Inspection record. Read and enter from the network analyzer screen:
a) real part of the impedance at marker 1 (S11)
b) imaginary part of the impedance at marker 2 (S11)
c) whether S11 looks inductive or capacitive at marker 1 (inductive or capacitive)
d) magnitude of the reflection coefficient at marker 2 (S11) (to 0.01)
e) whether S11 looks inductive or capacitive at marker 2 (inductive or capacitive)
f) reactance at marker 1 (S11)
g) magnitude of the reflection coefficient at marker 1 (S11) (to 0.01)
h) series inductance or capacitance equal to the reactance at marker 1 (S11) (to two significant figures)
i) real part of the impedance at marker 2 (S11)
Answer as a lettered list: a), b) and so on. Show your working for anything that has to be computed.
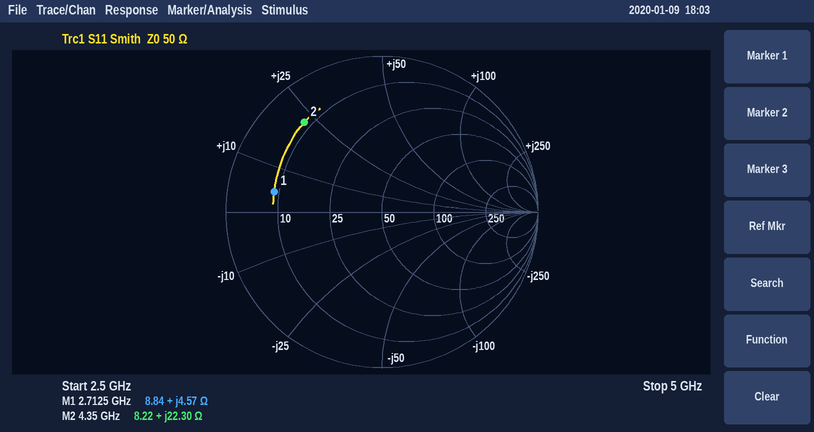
a) 8.84 Ω
b) +22.30 Ω
c) inductive
d) 0.76
e) inductive
f) +4.57 Ω
g) 0.70
h) L = 4.57 Ω/(2π × 2.7125 GHz) ≈ 268 pH, so 270 pH to two significant figures
i) 8.22 Ω
